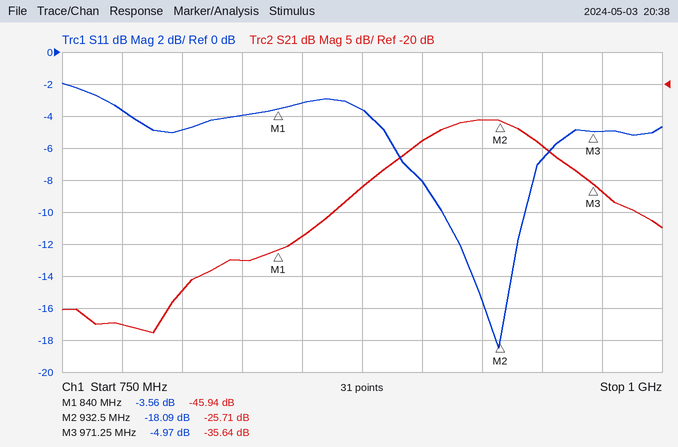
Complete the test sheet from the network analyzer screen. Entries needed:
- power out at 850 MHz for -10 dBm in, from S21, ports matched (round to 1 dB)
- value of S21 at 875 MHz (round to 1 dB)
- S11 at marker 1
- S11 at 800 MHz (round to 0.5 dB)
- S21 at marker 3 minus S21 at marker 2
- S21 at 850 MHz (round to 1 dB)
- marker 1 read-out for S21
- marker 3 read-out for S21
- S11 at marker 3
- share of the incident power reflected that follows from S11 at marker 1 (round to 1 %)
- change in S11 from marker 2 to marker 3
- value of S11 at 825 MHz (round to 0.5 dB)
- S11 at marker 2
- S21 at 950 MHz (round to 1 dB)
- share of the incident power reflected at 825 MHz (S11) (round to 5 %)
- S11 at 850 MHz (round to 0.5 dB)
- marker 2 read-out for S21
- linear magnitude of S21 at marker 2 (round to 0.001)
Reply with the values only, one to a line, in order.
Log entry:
-54 dBm
-36 dB
-3.56 dB
-5.0 dB
-9.93 dB
-44 dB
-45.94 dB
-35.64 dB
-4.97 dB
44 %
13.12 dB
-4.0 dB
-18.09 dB
-30 dB
40 %
-3.0 dB
-25.71 dB
0.052
